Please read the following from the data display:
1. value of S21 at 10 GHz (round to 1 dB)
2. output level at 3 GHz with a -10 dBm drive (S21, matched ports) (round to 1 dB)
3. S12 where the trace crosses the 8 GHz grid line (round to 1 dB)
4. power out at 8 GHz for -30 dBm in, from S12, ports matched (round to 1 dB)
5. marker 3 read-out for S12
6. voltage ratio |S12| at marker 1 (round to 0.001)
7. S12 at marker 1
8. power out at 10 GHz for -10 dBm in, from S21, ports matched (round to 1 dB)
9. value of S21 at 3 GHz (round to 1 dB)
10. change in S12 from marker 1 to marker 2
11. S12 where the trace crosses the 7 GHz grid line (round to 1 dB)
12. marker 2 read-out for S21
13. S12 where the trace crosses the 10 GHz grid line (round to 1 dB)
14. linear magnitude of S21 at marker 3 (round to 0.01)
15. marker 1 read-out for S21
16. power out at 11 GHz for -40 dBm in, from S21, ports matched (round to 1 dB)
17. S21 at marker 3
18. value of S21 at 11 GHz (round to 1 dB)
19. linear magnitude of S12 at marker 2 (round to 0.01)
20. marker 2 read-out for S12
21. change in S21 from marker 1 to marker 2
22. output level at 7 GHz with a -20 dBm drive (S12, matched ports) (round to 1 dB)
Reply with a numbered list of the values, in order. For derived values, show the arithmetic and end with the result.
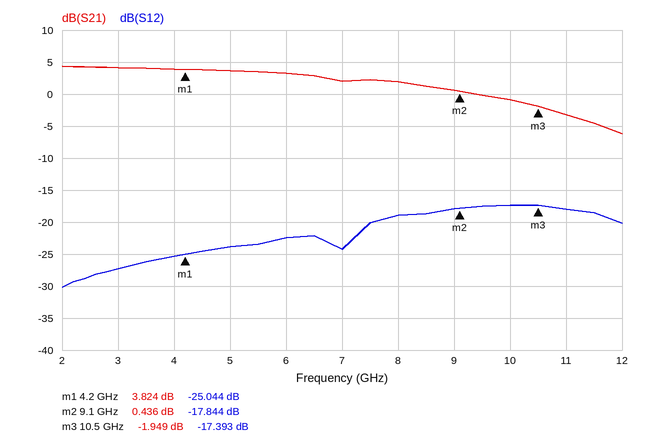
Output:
1. -1 dB
2. -10 dBm + (4 dB) = -6 dBm
3. -19 dB
4. -30 dBm + (-19 dB) = -49 dBm
5. -17.393 dB
6. 10^(-25.044/20) ≈ 0.056
7. -25.044 dB
8. -10 dBm + (-1 dB) = -11 dBm
9. 4 dB
10. -17.844 − (-25.044) = 7.200 dB
11. -24 dB
12. 0.436 dB
13. -17 dB
14. 10^(-1.949/20) ≈ 0.80
15. 3.824 dB
16. -40 dBm + (-3 dB) = -43 dBm
17. -1.949 dB
18. -3 dB
19. 10^(-17.844/20) ≈ 0.13
20. -17.844 dB
21. 0.436 − (3.824) = -3.388 dB
22. -20 dBm + (-24 dB) = -44 dBm
